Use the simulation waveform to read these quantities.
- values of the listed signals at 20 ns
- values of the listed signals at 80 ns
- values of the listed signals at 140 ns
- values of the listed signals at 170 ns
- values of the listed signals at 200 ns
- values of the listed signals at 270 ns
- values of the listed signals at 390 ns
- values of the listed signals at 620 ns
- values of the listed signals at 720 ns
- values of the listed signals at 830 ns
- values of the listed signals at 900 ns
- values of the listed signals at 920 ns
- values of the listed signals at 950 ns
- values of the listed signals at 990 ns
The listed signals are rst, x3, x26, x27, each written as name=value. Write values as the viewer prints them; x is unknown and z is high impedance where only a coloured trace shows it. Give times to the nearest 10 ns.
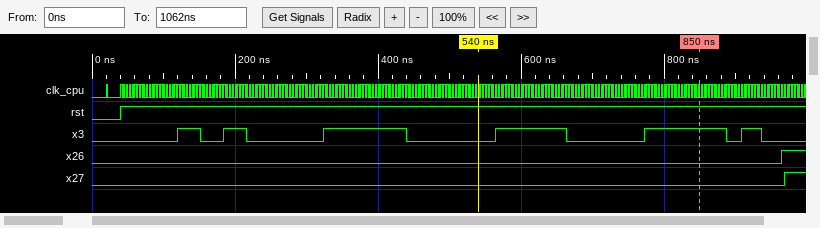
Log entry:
rst=0, x3=0, x26=0, x27=0
rst=1, x3=0, x26=0, x27=0
rst=1, x3=1, x26=0, x27=0
rst=1, x3=0, x26=0, x27=0
rst=1, x3=1, x26=0, x27=0
rst=1, x3=0, x26=0, x27=0
rst=1, x3=1, x26=0, x27=0
rst=1, x3=1, x26=0, x27=0
rst=1, x3=0, x26=0, x27=0
rst=1, x3=1, x26=0, x27=0
rst=1, x3=0, x26=0, x27=0
rst=1, x3=1, x26=0, x27=0
rst=1, x3=0, x26=0, x27=0
rst=1, x3=0, x26=1, x27=1
